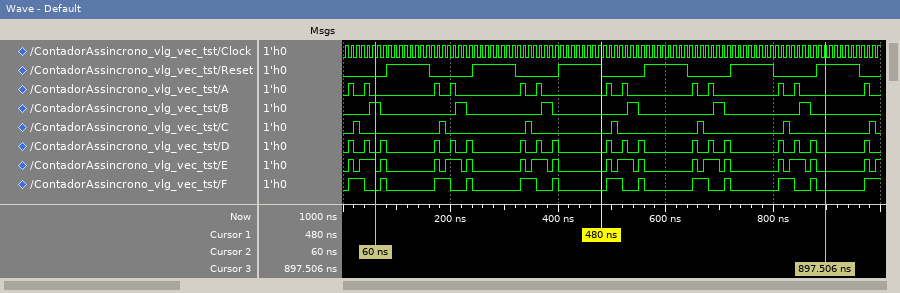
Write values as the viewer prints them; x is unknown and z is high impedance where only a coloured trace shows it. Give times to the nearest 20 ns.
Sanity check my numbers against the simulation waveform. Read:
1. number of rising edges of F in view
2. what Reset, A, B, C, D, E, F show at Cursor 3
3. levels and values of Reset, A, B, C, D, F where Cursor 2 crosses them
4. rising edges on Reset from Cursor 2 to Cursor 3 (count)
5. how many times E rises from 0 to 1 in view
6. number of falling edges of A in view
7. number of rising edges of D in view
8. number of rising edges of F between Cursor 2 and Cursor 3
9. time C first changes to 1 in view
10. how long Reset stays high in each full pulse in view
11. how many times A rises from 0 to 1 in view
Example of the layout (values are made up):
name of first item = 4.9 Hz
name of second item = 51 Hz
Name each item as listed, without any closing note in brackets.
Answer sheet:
number of rising edges of F in view = 13
what Reset, A, B, C, D, E, F show at Cursor 3 = Reset=1, A=0, B=0, C=0, D=0, E=0, F=0
levels and values of Reset, A, B, C, D, F where Cursor 2 crosses them = Reset=0, A=0, B=1, C=0, D=0, F=0
rising edges on Reset from Cursor 2 to Cursor 3 = 6
how many times E rises from 0 to 1 in view = 20
number of falling edges of A in view = 13
number of rising edges of D in view = 19
number of rising edges of F between Cursor 2 and Cursor 3 = 11
time C first changes to 1 in view = 20 ns
how long Reset stays high in each full pulse in view = 80 ns, 80 ns, 80 ns, 80 ns, 80 ns, 80 ns
how many times A rises from 0 to 1 in view = 13
